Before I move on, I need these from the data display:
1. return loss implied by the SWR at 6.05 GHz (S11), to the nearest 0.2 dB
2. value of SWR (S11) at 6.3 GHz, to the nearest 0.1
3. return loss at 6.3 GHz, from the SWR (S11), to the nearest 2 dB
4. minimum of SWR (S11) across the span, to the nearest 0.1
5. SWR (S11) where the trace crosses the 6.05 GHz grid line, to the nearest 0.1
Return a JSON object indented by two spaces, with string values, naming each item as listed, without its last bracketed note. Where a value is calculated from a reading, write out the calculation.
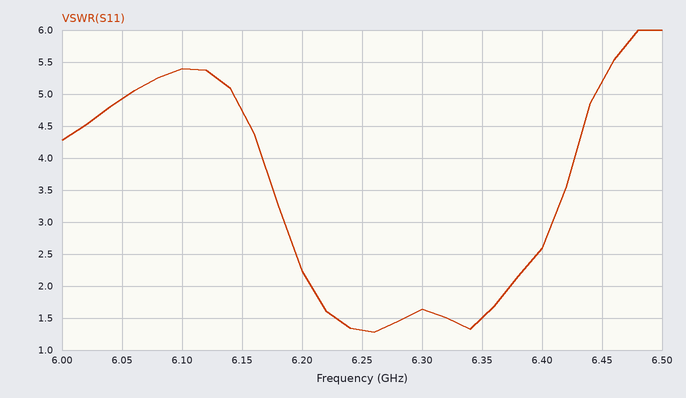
{
  "return loss implied by the SWR at 6.05 GHz (S11), to the nearest 0.2 dB": "−20 log10((4.9 − 1)/(4.9 + 1)) ≈ 3.6 dB",
  "value of SWR (S11) at 6.3 GHz, to the nearest 0.1": "1.6",
  "return loss at 6.3 GHz, from the SWR (S11), to the nearest 2 dB": "−20 log10((1.6 − 1)/(1.6 + 1)) ≈ 12.7 dB, so 12 dB to the nearest 2 dB",
  "minimum of SWR (S11) across the span, to the nearest 0.1": "1.3",
  "SWR (S11) where the trace crosses the 6.05 GHz grid line, to the nearest 0.1": "4.9"
}
